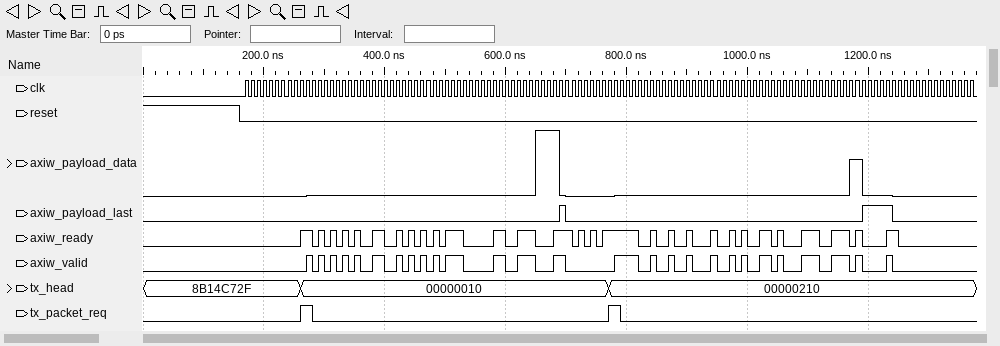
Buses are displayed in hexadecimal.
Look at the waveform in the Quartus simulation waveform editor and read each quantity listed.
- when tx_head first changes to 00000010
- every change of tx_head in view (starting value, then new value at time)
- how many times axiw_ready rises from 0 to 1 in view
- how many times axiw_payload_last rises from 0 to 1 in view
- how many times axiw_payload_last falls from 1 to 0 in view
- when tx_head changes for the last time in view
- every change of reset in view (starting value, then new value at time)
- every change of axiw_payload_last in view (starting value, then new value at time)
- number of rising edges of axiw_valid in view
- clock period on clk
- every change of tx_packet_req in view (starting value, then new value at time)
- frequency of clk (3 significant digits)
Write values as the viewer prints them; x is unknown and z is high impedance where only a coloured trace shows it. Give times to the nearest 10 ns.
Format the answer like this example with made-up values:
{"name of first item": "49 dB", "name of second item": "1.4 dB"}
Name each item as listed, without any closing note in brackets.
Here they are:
{"when tx_head first changes to 00000010": "260 ns", "every change of tx_head in view": "8B14C72F, 00000010 at 260 ns, 00000210 at 770 ns", "how many times axiw_ready rises from 0 to 1 in view": "29", "how many times axiw_payload_last rises from 0 to 1 in view": "2", "how many times axiw_payload_last falls from 1 to 0 in view": "2", "when tx_head changes for the last time in view": "770 ns", "every change of reset in view": "1, 0 at 160 ns", "every change of axiw_payload_last in view": "0, 1 at 690 ns, 0 at 700 ns, 1 at 1190 ns, 0 at 1240 ns", "number of rising edges of axiw_valid in view": "27", "clock period on clk": "10 ns", "every change of tx_packet_req in view": "0, 1 at 260 ns, 0 at 280 ns, 1 at 770 ns, 0 at 790 ns", "frequency of clk": "100 MHz"}
